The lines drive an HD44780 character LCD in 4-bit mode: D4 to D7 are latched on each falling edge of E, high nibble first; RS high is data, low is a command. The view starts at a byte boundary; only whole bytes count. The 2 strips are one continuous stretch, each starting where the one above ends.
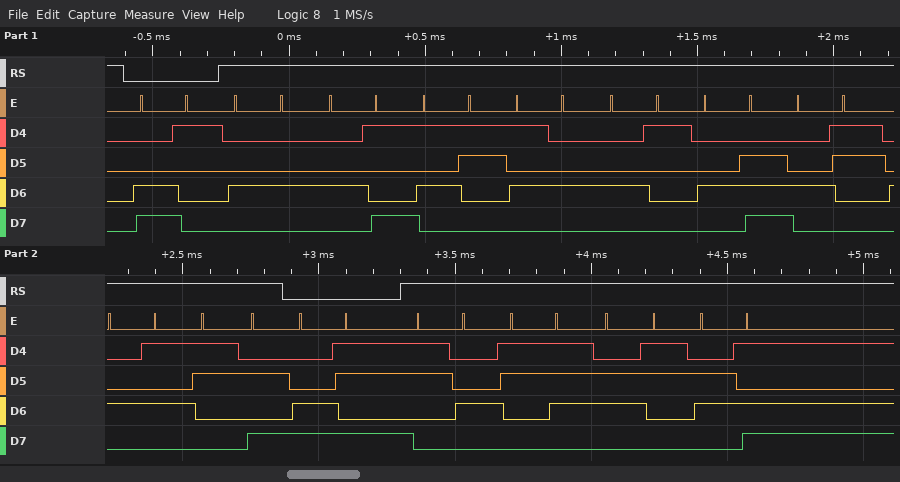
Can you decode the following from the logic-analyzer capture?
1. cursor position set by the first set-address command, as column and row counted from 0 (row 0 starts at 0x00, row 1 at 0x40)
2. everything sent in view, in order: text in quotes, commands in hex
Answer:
column 1, row 1
0xC1 "DISTANCE:" 0xCB "47cm"
